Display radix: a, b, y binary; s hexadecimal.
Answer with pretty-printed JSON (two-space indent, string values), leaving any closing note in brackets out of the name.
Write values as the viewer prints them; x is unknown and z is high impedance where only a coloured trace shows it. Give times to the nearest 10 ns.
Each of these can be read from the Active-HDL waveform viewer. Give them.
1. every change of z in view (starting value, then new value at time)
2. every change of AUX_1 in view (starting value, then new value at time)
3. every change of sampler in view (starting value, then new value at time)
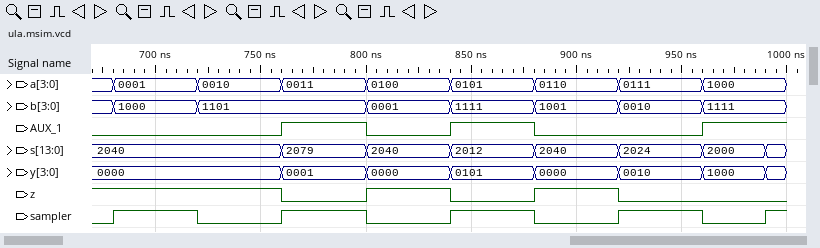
{
  "every change of z in view": "1, 0 at 760 ns, 1 at 800 ns, 0 at 840 ns, 1 at 880 ns, 0 at 920 ns",
  "every change of AUX_1 in view": "0, 1 at 760 ns, 0 at 800 ns, 1 at 840 ns, 0 at 880 ns, 1 at 960 ns",
  "every change of sampler in view": "0, 1 at 680 ns, 0 at 720 ns, 1 at 760 ns, 0 at 800 ns, 1 at 840 ns, 0 at 880 ns, 1 at 920 ns, 0 at 960 ns, 1 at 990 ns"
}
